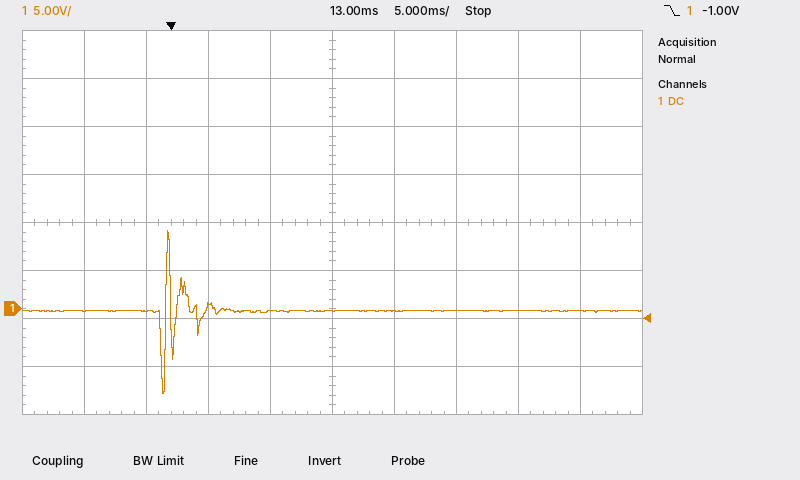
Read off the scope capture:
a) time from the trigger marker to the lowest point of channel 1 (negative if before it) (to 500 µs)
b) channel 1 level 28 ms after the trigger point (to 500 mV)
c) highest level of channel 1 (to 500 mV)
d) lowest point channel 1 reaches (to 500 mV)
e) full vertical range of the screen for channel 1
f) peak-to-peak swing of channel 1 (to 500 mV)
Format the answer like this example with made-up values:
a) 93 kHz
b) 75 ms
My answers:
a) -500 µs
b) 0.0 V
c) 8.0 V
d) -9.0 V
e) 40 V
f) 17.0 V
